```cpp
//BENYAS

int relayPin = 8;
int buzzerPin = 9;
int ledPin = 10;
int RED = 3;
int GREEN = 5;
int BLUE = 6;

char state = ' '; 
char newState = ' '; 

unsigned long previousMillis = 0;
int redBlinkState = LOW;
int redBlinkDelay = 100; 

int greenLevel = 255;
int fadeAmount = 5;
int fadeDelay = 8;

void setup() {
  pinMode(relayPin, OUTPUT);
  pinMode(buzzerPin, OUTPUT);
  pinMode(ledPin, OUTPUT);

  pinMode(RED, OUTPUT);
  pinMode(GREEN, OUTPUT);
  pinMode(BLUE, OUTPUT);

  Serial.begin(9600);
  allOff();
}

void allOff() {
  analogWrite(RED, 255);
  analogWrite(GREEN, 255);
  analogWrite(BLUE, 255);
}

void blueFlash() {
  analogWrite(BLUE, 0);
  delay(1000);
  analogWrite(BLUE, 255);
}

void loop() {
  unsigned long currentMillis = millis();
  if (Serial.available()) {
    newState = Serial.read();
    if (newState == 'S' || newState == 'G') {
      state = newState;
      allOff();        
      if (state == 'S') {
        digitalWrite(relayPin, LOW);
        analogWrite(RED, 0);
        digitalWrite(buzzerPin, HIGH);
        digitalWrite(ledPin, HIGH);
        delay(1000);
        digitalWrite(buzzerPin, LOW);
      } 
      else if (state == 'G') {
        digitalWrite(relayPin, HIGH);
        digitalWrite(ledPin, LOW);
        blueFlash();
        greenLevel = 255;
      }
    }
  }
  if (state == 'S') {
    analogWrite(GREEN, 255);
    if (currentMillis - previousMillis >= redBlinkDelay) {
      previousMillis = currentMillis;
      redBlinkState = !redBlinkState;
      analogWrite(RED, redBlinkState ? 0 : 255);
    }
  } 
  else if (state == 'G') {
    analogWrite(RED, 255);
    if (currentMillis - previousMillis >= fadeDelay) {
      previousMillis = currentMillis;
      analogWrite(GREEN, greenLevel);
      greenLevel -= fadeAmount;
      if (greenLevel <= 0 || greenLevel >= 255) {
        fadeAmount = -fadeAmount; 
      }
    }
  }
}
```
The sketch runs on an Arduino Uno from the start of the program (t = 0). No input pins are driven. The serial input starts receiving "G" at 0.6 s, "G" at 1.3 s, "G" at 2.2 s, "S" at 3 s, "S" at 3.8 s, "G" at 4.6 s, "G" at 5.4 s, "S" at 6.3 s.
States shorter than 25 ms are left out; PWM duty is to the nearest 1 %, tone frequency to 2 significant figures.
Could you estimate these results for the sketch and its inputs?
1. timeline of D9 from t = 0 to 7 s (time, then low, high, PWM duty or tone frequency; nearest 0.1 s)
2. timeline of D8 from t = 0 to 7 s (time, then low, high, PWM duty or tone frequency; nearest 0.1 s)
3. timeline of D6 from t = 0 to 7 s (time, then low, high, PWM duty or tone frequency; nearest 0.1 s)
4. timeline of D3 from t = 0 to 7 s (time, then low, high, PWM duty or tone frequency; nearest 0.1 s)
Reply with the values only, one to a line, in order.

0 s low; 3.6 s high; 5.6 s low
0 s low; 0.6 s high; 3.6 s low; 5.6 s high
0 s high; 0.6 s low; 3.6 s high; 5.6 s low
0 s high; 3.6 s low; 5.6 s high
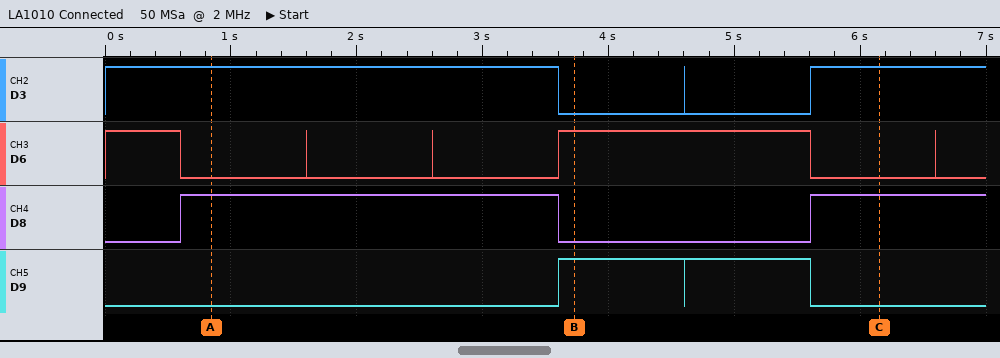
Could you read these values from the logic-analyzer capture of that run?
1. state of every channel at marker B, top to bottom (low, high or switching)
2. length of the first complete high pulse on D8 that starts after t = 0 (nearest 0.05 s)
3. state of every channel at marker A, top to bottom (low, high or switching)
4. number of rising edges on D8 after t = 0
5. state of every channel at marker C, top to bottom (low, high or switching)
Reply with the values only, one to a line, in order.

D3 low, D6 high, D8 low, D9 high
3.00 s
D3 high, D6 low, D8 high, D9 low
2
D3 high, D6 low, D8 high, D9 low
